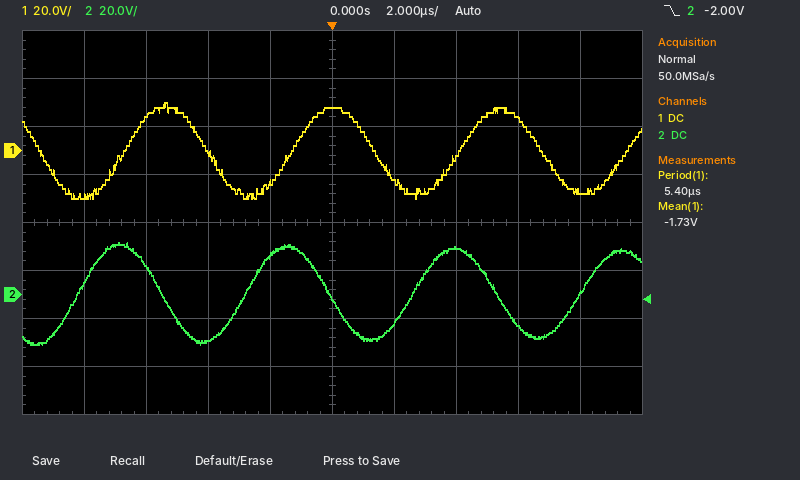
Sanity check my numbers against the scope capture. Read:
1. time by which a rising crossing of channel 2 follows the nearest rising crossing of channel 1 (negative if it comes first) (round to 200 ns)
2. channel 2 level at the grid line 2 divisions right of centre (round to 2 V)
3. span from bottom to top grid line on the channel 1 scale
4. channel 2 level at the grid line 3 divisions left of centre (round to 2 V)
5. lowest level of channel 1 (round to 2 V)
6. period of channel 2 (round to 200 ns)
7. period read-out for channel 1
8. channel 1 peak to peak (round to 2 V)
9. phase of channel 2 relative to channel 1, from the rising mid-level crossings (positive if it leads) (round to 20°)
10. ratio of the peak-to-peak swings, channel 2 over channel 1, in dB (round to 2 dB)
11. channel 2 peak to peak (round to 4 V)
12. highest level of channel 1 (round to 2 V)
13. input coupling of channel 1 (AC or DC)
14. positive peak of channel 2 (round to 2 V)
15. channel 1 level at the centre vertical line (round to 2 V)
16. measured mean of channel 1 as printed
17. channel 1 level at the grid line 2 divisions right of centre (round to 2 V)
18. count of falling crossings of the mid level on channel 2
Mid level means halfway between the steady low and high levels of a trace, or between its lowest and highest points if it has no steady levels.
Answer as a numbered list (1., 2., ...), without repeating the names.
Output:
1. -1.6 µs
2. 20 V
3. 160 V
4. 12 V
5. -20 V
6. 5.4 µs
7. 5.40 µs
8. 40 V
9. +100°
10. 0 dB
11. 44 V
12. 20 V
13. DC
14. 22 V
15. 18 V
16. -1.73 V
17. -2 V
18. 3
